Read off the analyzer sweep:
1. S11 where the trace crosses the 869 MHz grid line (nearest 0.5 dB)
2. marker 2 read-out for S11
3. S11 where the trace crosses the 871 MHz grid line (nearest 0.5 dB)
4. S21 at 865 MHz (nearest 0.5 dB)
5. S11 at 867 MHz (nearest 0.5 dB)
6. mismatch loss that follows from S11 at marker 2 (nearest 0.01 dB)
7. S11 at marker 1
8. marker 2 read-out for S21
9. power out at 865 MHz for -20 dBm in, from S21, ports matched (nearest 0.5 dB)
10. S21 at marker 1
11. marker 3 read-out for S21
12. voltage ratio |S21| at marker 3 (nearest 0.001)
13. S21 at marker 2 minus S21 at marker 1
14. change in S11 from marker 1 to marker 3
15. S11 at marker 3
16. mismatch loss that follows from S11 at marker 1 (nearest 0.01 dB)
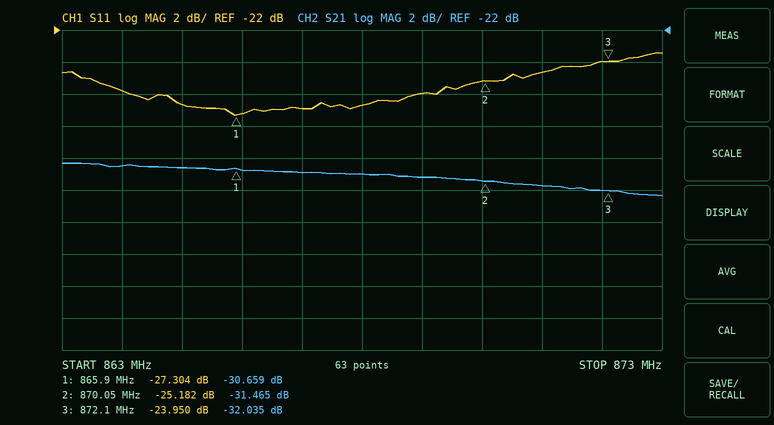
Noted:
-26.0 dB
-25.182 dB
-24.5 dB
-30.5 dB
-27.0 dB
0.01 dB
-27.304 dB
-31.465 dB
-50.5 dBm
-30.659 dB
-32.035 dB
0.025
-0.806 dB
3.354 dB
-23.950 dB
0.01 dB
